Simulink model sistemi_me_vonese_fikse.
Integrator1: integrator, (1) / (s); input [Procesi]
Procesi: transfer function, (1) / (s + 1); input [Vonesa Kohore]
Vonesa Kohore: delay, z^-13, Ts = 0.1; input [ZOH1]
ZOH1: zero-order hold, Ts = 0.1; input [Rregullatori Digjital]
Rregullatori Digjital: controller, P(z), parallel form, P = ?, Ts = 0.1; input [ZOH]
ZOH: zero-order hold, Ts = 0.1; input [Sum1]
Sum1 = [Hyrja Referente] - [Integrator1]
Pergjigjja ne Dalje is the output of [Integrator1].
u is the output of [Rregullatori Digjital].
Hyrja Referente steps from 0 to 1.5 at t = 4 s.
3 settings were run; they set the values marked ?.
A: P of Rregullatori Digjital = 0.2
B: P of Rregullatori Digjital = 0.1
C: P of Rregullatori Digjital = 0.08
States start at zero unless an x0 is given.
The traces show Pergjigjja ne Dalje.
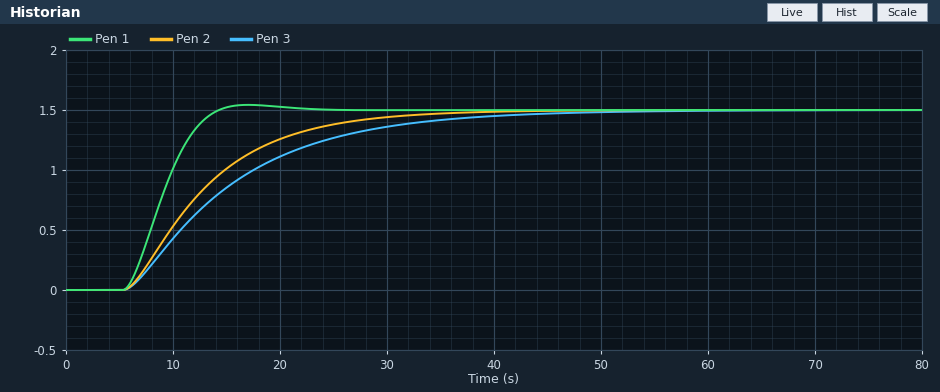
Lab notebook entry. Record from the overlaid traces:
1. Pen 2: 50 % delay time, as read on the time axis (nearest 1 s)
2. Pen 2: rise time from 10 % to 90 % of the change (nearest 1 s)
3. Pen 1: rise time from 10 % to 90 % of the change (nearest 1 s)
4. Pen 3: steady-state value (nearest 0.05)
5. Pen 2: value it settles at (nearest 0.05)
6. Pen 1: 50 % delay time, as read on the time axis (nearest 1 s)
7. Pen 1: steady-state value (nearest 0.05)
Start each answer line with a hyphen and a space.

- 12 s
- 16 s
- 6 s
- 1.50
- 1.50
- 9 s
- 1.50
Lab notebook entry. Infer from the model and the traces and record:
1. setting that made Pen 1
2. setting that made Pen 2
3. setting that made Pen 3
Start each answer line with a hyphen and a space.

- A
- B
- C
